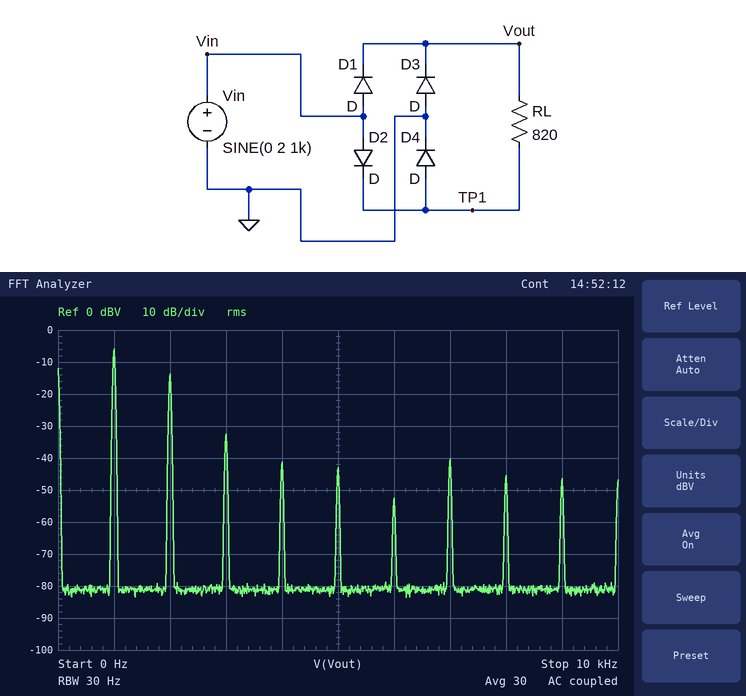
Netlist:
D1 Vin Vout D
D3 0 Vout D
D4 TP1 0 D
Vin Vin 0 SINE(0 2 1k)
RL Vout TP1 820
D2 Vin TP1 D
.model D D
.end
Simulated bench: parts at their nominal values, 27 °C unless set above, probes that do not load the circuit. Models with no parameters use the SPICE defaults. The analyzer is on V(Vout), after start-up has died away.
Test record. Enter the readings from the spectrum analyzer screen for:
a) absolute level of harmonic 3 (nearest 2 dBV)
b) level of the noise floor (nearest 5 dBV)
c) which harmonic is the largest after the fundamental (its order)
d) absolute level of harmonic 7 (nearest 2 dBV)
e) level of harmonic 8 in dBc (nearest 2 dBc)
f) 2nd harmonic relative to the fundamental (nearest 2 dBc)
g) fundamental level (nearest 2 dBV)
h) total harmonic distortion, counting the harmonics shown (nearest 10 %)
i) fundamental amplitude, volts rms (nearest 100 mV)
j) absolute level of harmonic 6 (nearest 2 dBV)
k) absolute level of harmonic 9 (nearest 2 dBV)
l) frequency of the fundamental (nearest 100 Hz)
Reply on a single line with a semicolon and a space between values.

-32 dBV; -80 dBV; 2; -40 dBV; -40 dBc; -8 dBc; -6 dBV; 40 %; 500 mV; -52 dBV; -46 dBV; 1.0 kHz
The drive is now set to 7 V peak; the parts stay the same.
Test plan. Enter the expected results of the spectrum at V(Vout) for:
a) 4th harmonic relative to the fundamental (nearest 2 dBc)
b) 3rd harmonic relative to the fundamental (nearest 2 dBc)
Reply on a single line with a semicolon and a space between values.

-22 dBc; -30 dBc
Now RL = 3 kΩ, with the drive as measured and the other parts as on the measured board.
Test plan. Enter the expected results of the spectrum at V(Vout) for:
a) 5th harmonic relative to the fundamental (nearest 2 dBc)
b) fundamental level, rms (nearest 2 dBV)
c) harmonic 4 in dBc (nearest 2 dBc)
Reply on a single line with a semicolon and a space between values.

-40 dBc; -6 dBV; -34 dBc
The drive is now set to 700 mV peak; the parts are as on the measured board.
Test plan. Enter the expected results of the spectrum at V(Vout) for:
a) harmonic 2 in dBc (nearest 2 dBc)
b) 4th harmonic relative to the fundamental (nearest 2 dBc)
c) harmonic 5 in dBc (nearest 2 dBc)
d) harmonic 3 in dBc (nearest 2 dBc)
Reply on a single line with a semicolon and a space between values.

-12 dBc; -30 dBc; -34 dBc; -26 dBc
